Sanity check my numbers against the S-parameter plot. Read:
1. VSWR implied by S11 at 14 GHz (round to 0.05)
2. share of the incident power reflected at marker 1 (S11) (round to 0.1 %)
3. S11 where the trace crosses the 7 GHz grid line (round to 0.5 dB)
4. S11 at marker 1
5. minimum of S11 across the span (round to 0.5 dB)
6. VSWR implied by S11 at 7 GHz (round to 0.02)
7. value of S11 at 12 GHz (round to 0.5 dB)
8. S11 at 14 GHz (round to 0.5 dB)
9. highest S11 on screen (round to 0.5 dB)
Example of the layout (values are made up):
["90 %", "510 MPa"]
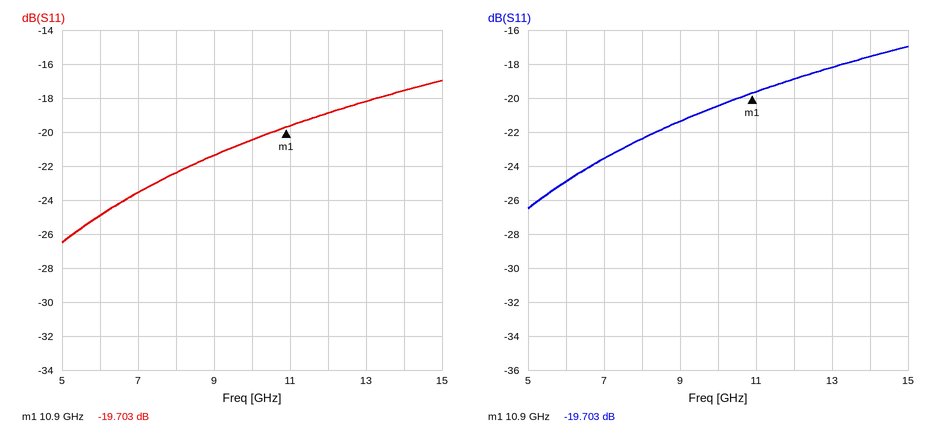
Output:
["1.30", "1.1 %", "-23.5 dB", "-19.703 dB", "-26.5 dB", "1.14", "-19.0 dB", "-17.5 dB", "-17.0 dB"]
